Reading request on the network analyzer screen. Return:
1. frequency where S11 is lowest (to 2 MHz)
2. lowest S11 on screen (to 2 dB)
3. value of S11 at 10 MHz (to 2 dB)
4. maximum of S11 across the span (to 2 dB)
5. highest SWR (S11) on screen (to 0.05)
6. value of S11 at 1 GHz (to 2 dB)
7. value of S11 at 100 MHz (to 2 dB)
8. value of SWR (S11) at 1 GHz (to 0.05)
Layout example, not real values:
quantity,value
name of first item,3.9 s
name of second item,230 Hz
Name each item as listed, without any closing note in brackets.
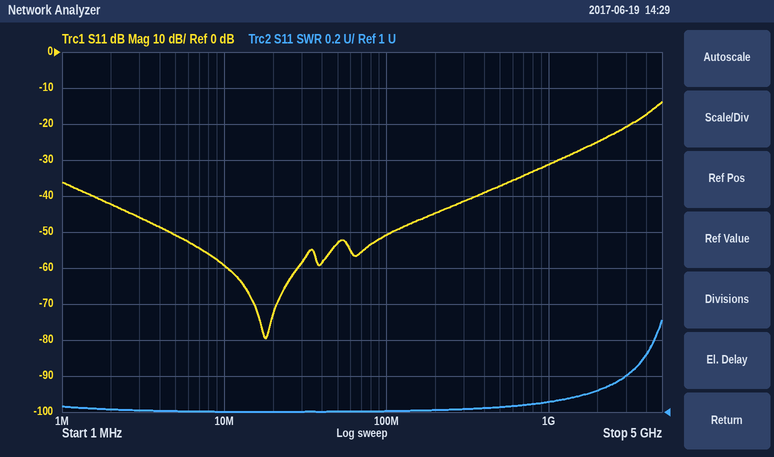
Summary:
quantity,value
frequency where S11 is lowest,18 MHz
lowest S11 on screen,-80 dB
value of S11 at 10 MHz,-60 dB
maximum of S11 across the span,-14 dB
highest SWR (S11) on screen,1.50
value of S11 at 1 GHz,-32 dB
value of S11 at 100 MHz,-50 dB
value of SWR (S11) at 1 GHz,1.05
